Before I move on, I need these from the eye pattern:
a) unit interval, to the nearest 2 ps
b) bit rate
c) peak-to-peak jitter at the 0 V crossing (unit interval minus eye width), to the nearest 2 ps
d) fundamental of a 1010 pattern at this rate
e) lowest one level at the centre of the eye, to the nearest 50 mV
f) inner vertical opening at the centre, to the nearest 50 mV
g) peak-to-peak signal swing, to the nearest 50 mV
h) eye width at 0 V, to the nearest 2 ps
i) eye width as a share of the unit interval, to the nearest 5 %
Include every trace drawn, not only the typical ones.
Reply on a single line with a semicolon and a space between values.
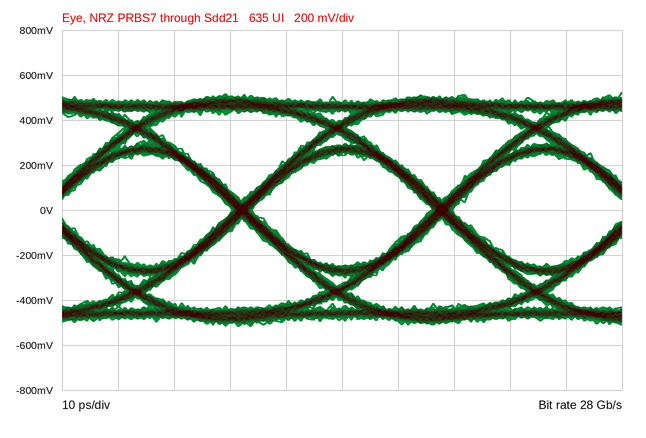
36 ps; 28 Gb/s; 4 ps; 14 GHz; 250 mV; 500 mV; 1.05 V; 32 ps; 90 %
